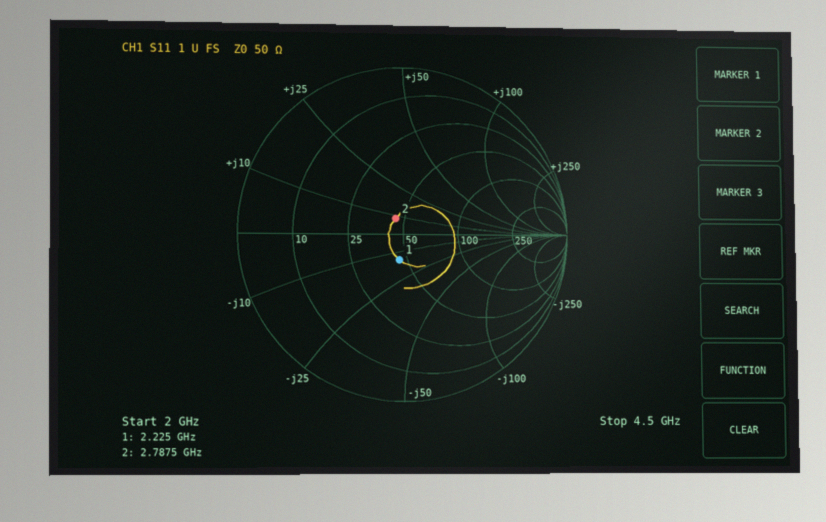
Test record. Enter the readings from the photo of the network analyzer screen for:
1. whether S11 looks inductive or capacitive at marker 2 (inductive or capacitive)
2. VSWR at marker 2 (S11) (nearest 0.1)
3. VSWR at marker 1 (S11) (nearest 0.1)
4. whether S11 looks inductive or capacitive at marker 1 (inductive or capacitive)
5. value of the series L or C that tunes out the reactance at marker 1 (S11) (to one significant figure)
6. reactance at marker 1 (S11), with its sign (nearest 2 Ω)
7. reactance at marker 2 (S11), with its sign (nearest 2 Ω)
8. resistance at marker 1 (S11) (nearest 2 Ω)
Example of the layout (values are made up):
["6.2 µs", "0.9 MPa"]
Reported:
["inductive", "1.2", "1.4", "capacitive", "1 nH", "-14 Ω", "+8 Ω", "46 Ω"]
